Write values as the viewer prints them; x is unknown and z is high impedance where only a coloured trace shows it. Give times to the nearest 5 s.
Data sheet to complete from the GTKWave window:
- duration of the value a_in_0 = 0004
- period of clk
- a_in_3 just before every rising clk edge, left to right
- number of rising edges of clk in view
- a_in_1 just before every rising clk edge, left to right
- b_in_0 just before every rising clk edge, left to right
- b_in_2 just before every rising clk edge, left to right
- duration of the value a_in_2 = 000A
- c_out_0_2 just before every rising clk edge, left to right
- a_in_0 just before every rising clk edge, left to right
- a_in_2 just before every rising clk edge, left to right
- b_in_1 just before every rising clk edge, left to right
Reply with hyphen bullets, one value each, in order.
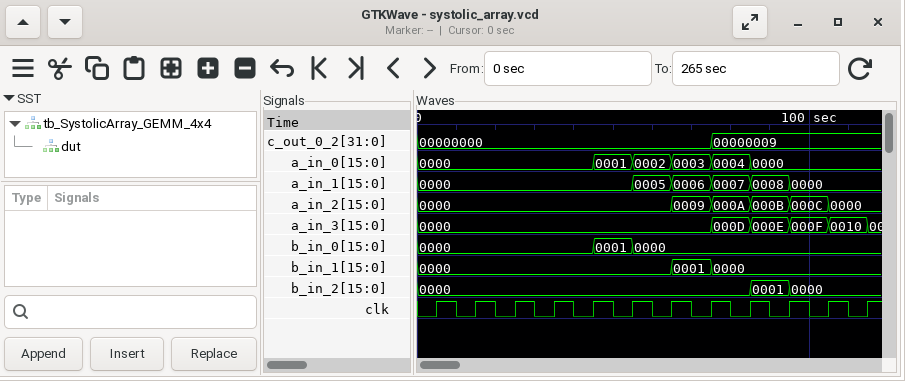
- 10 s
- 10 s
- 0000, 0000, 0000, 0000, 0000, 0000, 0000, 0000, 000D, 000E, 000F, 0010
- 12
- 0000, 0000, 0000, 0000, 0000, 0000, 0005, 0006, 0007, 0008, 0000, 0000
- 0000, 0000, 0000, 0000, 0000, 0001, 0000, 0000, 0000, 0000, 0000, 0000
- 0000, 0000, 0000, 0000, 0000, 0000, 0000, 0000, 0000, 0001, 0000, 0000
- 10 s
- 00000000, 00000000, 00000000, 00000000, 00000000, 00000000, 00000000, 00000000, 00000009, 00000009, 00000009, 00000009
- 0000, 0000, 0000, 0000, 0000, 0001, 0002, 0003, 0004, 0000, 0000, 0000
- 0000, 0000, 0000, 0000, 0000, 0000, 0000, 0009, 000A, 000B, 000C, 0000
- 0000, 0000, 0000, 0000, 0000, 0000, 0000, 0001, 0000, 0000, 0000, 0000
